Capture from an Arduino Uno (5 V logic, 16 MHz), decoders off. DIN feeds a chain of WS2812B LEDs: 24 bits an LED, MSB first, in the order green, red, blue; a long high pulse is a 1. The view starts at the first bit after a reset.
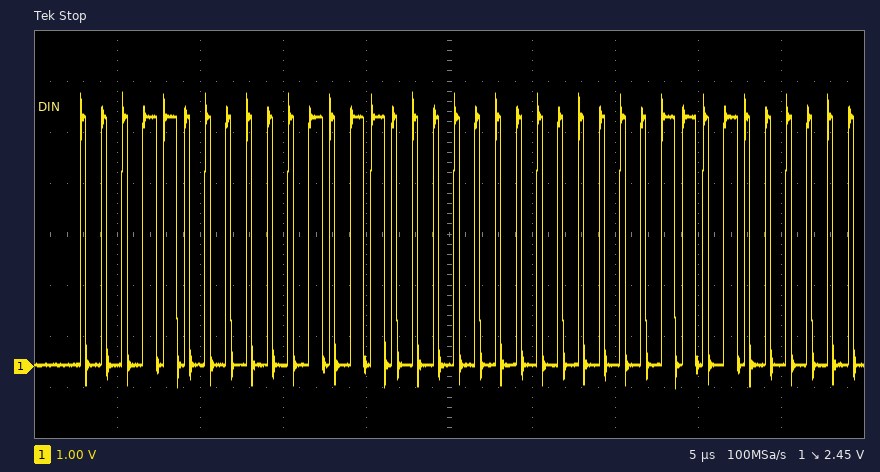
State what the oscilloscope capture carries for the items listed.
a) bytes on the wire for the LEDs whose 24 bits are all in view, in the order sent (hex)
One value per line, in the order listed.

18 16 00
